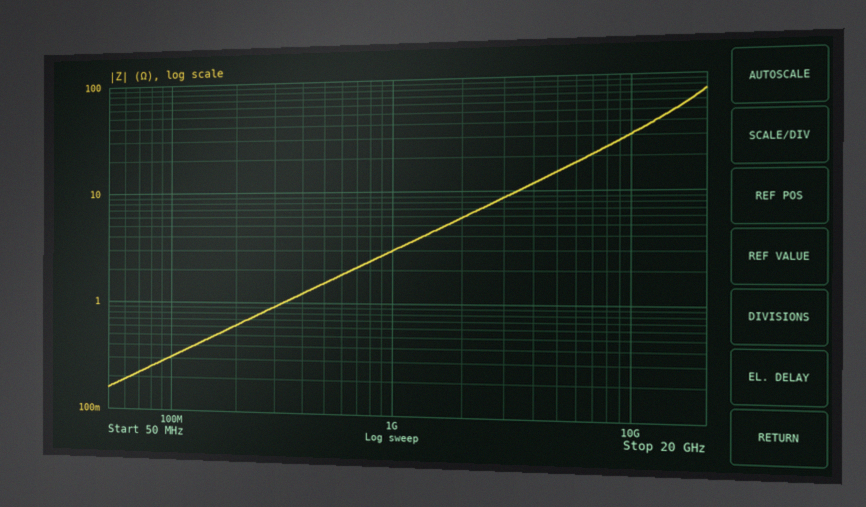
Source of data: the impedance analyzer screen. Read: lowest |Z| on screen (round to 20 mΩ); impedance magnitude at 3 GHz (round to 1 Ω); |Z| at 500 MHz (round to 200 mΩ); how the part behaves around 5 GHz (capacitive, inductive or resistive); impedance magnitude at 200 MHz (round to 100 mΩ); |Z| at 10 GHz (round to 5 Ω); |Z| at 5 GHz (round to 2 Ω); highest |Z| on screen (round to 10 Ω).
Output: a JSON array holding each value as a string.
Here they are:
["160 mΩ", "9 Ω", "1.6 Ω", "inductive", "600 mΩ", "30 Ω", "14 Ω", "70 Ω"]
